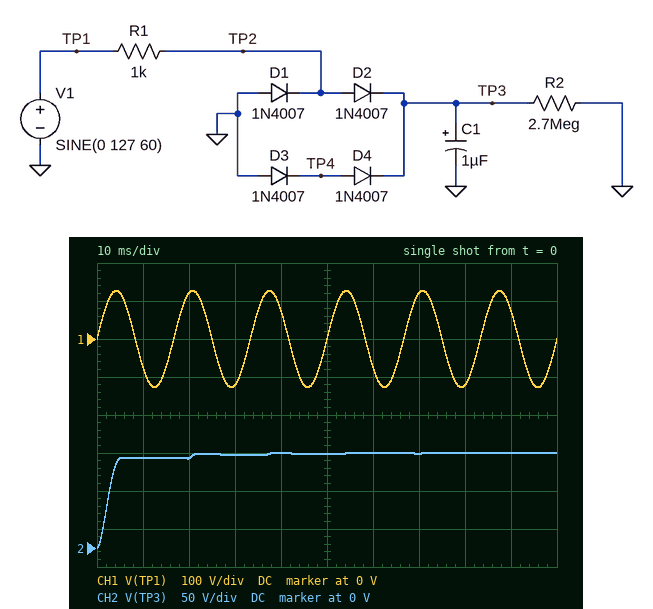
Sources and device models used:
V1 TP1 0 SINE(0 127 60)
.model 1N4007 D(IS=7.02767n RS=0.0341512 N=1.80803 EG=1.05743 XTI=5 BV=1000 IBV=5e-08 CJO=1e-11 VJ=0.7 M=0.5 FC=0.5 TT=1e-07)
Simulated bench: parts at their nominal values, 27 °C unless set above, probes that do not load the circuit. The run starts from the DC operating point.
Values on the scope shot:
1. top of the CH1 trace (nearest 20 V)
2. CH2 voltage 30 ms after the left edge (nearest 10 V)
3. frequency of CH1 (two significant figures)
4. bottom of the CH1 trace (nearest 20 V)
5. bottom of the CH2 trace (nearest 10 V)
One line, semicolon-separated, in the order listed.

120 V; 120 V; 60 Hz; -120 V; 0 V
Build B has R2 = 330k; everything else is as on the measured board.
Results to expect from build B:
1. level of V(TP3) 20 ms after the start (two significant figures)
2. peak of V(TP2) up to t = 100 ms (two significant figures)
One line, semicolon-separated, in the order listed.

110 V; 120 V
